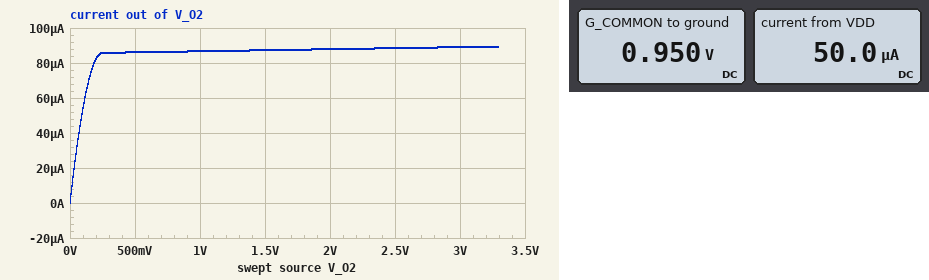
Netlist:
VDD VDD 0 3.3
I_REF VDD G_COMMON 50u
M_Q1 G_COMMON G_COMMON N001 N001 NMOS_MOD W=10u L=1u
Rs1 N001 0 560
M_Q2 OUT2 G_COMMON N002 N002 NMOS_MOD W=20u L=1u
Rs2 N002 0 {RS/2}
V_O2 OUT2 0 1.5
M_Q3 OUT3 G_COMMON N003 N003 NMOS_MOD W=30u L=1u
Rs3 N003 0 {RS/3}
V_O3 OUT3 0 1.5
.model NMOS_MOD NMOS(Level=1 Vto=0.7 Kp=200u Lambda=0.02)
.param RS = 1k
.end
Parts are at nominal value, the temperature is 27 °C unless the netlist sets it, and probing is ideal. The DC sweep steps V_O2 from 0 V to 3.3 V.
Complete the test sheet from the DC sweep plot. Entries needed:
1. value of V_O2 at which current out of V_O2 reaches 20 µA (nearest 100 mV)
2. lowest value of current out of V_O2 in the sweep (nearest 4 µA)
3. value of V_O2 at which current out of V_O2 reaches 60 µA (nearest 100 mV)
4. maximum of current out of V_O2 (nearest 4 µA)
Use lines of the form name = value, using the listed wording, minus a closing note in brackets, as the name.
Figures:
value of V_O2 at which current out of V_O2 reaches 20 µA = 0 V
lowest value of current out of V_O2 in the sweep = 0 A
value of V_O2 at which current out of V_O2 reaches 60 µA = 100 mV
maximum of current out of V_O2 = 88 µA
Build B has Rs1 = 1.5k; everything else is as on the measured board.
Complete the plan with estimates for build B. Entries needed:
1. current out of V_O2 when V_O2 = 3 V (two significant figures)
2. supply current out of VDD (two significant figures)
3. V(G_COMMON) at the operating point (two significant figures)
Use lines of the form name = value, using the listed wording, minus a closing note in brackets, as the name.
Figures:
current out of V_O2 when V_O2 = 3 V = 120 µA
supply current out of VDD = 50 µA
V(G_COMMON) at the operating point = 1.0 V
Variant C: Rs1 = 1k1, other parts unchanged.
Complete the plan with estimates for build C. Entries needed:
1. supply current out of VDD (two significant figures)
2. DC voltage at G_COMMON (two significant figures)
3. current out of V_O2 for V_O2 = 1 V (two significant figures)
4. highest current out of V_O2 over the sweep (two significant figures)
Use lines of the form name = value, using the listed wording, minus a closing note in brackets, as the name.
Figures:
supply current out of VDD = 50 µA
DC voltage at G_COMMON = 980 mV
current out of V_O2 for V_O2 = 1 V = 100 µA
highest current out of V_O2 over the sweep = 110 µA
